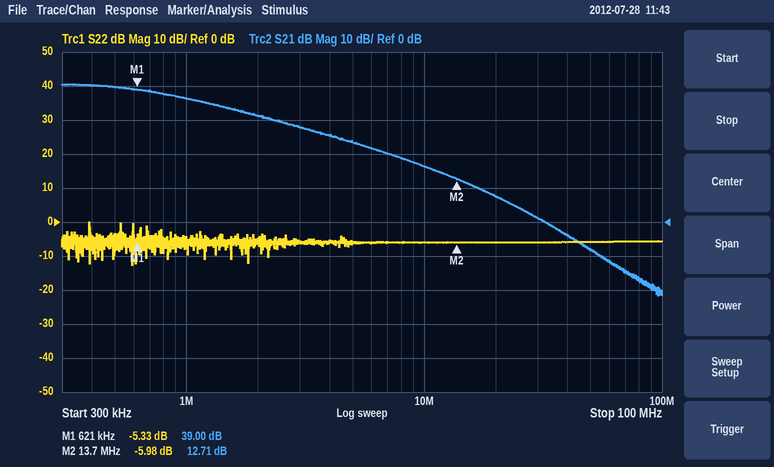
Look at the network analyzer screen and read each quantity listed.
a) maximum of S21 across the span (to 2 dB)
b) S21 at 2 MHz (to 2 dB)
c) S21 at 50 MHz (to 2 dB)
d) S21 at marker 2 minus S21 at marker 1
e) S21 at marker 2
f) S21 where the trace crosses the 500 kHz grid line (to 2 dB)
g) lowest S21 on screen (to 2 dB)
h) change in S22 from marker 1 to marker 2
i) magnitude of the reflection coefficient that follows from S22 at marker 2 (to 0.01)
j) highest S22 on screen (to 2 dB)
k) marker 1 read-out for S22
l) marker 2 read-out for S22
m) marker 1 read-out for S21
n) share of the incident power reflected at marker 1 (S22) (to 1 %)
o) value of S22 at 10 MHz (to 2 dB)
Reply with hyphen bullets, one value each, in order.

- 40 dB
- 32 dB
- -8 dB
- -26.29 dB
- 12.71 dB
- 40 dB
- -22 dB
- -0.65 dB
- 0.50
- 0 dB
- -5.33 dB
- -5.98 dB
- 39.00 dB
- 29 %
- -6 dB
